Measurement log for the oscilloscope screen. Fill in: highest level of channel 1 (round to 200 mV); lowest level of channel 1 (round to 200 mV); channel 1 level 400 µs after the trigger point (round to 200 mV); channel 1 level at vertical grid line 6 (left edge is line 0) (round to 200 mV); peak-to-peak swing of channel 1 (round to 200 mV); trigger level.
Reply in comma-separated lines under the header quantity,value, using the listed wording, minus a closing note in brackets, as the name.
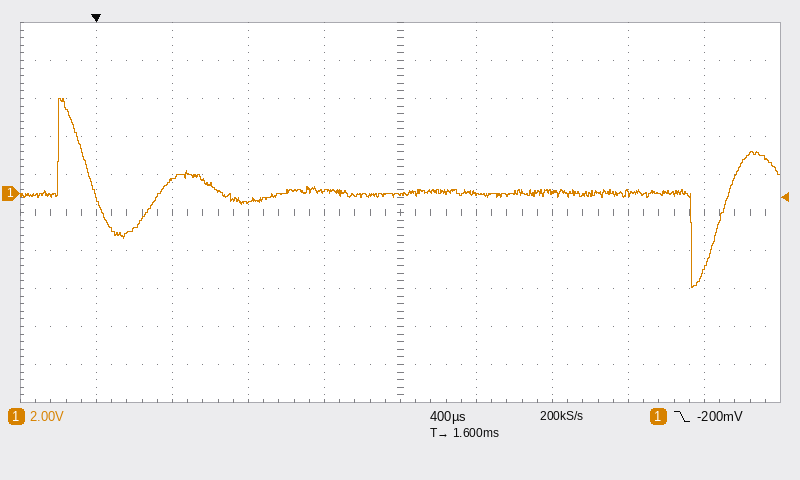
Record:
quantity,value
highest level of channel 1,5.0 V
lowest level of channel 1,-5.0 V
channel 1 level 400 µs after the trigger point,800 mV
channel 1 level at vertical grid line 6 (left edge is line 0),0.0 V
peak-to-peak swing of channel 1,10.0 V
trigger level,-200 mV
